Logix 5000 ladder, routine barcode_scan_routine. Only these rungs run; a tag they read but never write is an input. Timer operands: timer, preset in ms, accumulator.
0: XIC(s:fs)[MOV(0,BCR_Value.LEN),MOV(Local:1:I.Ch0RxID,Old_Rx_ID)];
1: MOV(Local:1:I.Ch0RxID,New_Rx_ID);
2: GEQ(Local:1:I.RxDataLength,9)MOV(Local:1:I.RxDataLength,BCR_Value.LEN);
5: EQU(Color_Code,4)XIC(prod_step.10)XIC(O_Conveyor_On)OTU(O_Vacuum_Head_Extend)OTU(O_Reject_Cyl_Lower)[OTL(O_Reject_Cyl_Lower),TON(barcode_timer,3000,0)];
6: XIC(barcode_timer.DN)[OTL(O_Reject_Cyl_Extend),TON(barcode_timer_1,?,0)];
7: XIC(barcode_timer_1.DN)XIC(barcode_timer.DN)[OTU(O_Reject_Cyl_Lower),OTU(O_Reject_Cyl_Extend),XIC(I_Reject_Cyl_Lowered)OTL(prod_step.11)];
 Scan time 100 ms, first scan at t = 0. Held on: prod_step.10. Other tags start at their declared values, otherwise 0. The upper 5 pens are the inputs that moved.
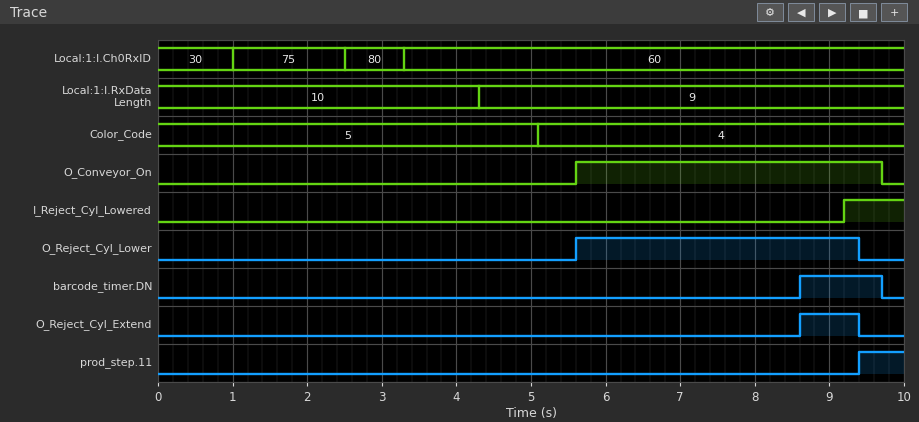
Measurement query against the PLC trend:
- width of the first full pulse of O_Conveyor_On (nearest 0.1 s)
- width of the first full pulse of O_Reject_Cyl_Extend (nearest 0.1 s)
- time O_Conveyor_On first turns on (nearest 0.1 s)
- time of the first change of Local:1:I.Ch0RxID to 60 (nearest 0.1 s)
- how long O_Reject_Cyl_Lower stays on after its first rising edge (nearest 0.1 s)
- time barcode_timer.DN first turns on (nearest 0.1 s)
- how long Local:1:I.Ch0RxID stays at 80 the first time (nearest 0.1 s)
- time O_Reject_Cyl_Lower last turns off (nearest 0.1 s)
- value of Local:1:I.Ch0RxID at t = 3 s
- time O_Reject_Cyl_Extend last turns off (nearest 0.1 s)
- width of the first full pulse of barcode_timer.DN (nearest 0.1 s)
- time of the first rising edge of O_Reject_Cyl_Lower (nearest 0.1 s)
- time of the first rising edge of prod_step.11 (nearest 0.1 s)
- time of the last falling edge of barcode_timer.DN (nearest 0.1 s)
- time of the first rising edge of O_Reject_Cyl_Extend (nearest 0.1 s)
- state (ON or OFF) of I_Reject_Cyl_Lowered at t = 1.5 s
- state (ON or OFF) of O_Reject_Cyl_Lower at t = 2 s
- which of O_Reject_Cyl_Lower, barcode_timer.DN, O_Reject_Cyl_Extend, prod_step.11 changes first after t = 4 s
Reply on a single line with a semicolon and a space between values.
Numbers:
4.1 s; 0.8 s; 5.6 s; 3.3 s; 3.8 s; 8.6 s; 0.8 s; 9.4 s; 80; 9.4 s; 1.1 s; 5.6 s; 9.4 s; 9.7 s; 8.6 s; OFF; OFF; O_Reject_Cyl_Lower
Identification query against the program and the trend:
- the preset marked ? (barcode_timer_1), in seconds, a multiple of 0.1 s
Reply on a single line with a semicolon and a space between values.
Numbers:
0.8 s
